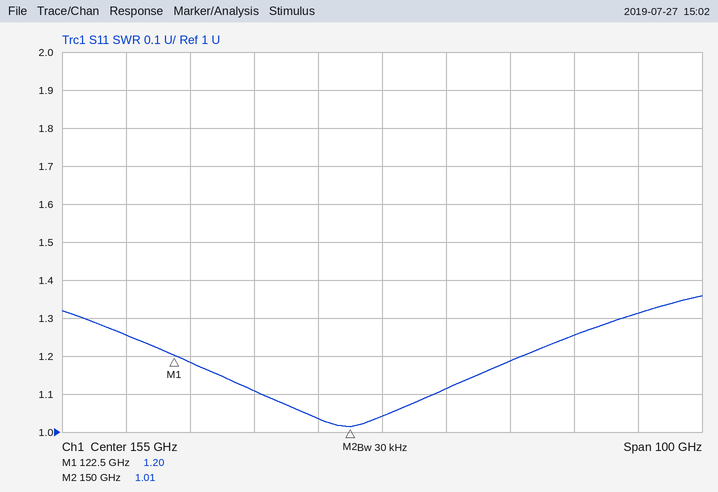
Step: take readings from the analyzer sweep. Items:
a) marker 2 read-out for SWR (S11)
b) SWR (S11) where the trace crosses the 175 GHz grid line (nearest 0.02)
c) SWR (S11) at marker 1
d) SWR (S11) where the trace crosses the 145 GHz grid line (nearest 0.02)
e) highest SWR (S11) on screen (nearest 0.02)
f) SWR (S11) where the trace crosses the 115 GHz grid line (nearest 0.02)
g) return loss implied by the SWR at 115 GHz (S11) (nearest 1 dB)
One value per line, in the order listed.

1.01
1.18
1.20
1.04
1.36
1.26
19 dB
